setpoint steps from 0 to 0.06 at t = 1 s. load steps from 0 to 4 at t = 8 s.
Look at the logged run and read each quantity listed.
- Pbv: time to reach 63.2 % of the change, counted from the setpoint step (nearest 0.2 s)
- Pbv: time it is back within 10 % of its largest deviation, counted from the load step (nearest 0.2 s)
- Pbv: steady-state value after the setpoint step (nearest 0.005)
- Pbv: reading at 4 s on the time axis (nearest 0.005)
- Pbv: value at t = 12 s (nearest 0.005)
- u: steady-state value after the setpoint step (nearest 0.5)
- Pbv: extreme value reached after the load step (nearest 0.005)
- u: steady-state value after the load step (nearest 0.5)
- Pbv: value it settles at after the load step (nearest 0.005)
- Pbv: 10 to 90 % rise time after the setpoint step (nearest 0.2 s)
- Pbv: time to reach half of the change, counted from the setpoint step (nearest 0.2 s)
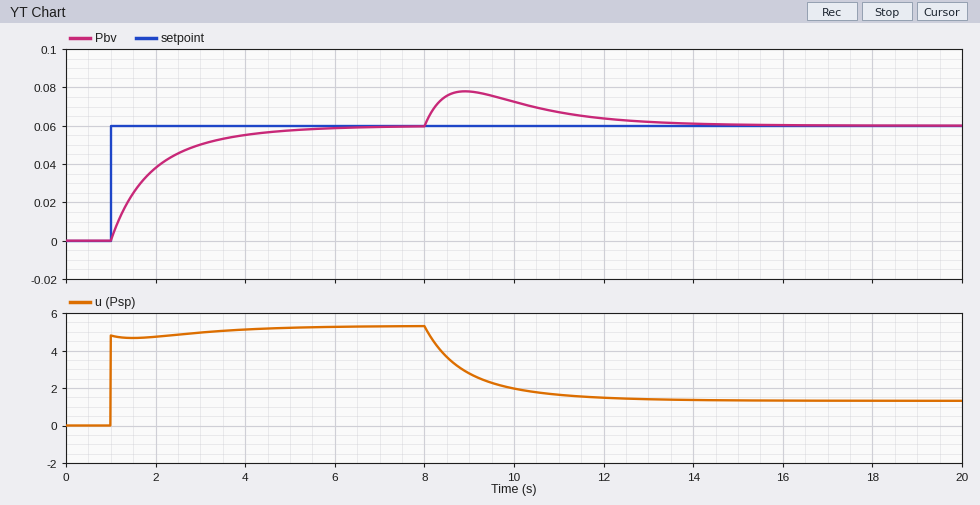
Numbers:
1.0 s
5.2 s
0.060
0.055
0.065
5.5
0.080
1.5
0.060
2.6 s
0.6 s
